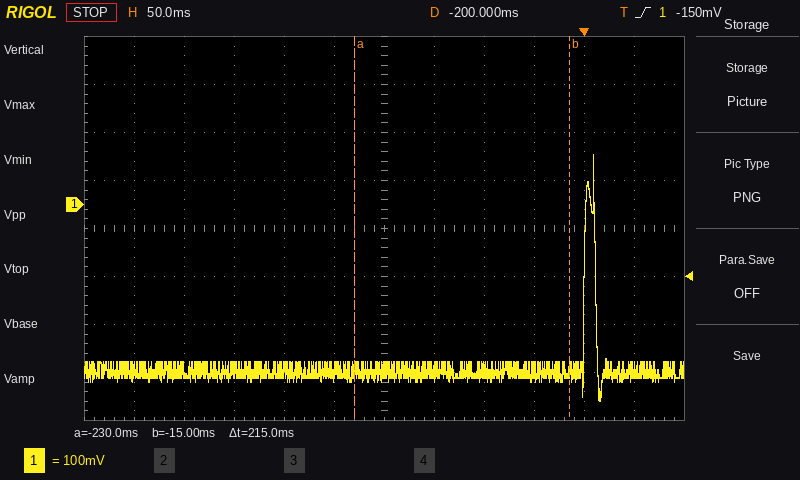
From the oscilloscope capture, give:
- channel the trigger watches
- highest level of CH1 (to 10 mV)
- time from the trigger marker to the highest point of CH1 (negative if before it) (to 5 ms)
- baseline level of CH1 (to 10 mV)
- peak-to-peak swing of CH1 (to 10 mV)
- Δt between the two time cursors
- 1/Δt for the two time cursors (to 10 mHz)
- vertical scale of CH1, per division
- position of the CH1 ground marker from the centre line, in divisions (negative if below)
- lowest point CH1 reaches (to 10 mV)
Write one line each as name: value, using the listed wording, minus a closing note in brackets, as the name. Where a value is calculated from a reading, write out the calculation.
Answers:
channel the trigger watches: CH1
highest level of CH1: 100 mV
time from the trigger marker to the highest point of CH1 (negative if before it): +10 ms
baseline level of CH1: -340 mV
peak-to-peak swing of CH1: 100 mV − (-410 mV) = 510 mV
Δt between the two time cursors: 215 ms
1/Δt for the two time cursors: 1 / 215 ms ≈ 4.65 Hz
vertical scale of CH1, per division: 100 mV
position of the CH1 ground marker from the centre line, in divisions: +0.5 div
lowest point CH1 reaches: -410 mV
